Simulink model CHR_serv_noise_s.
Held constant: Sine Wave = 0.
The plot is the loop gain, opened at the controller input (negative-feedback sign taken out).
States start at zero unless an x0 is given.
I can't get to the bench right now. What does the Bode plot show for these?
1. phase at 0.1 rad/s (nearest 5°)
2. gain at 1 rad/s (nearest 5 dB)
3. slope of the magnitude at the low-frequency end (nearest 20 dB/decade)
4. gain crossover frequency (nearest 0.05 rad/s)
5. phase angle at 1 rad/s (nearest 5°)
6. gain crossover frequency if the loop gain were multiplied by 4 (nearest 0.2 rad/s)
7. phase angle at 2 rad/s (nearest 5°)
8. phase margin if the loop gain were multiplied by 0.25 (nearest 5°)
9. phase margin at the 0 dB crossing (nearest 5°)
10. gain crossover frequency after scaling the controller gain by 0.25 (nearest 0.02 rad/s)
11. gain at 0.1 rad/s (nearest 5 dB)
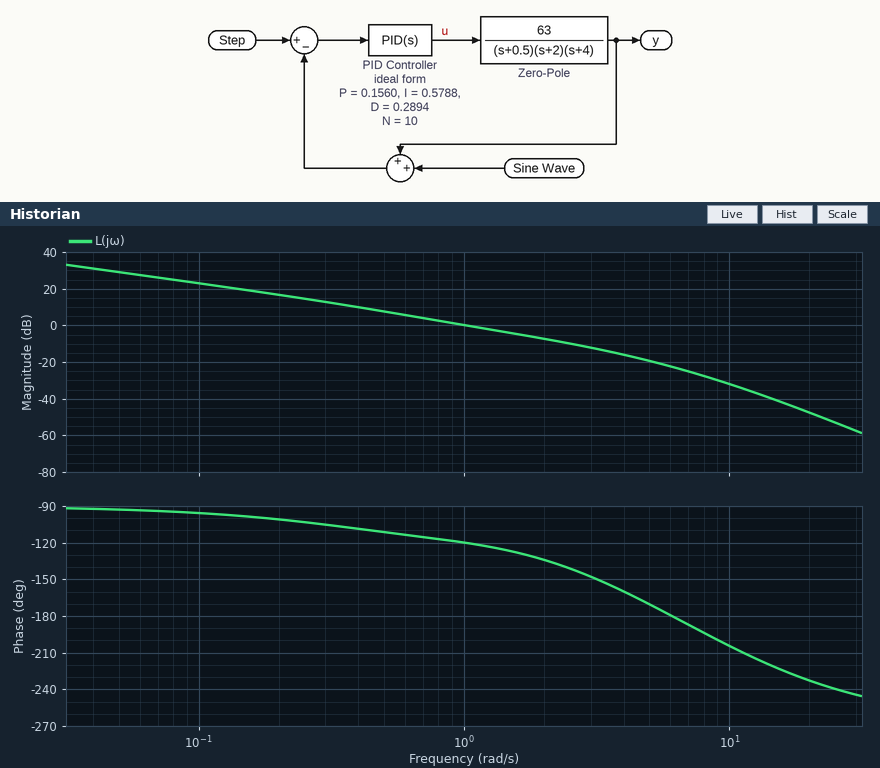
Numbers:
-95°
0 dB
-20 dB/decade
1.00 rad/s
-120°
3.0 rad/s
-135°
75°
60°
0.32 rad/s
25 dB
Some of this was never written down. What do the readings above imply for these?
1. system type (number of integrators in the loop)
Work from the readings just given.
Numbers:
1
